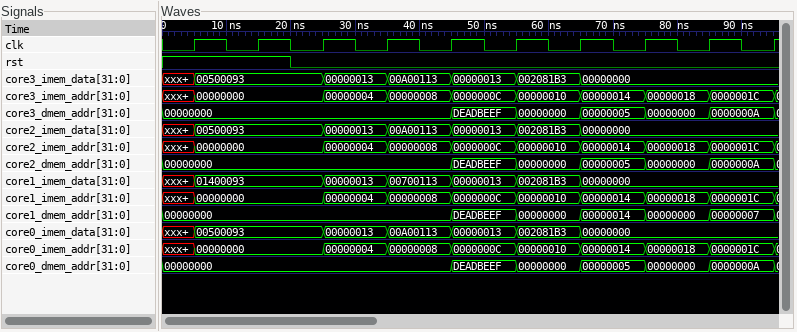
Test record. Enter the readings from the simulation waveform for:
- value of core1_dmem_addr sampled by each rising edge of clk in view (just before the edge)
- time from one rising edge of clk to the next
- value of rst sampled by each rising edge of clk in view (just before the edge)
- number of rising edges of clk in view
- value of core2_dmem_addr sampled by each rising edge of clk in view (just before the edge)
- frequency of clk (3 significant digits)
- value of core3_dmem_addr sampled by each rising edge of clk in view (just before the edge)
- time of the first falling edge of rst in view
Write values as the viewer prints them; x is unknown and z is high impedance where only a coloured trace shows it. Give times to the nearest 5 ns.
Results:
00000000, 00000000, 00000000, 00000000, 00000000, DEADBEEF, 00000000, 00000014, 00000000, 00000007
10 ns
1 1 0 0 0 0 0 0 0 0
10
00000000, 00000000, 00000000, 00000000, 00000000, DEADBEEF, 00000000, 00000005, 00000000, 0000000A
100 MHz
00000000, 00000000, 00000000, 00000000, 00000000, DEADBEEF, 00000000, 00000005, 00000000, 0000000A
20 ns
